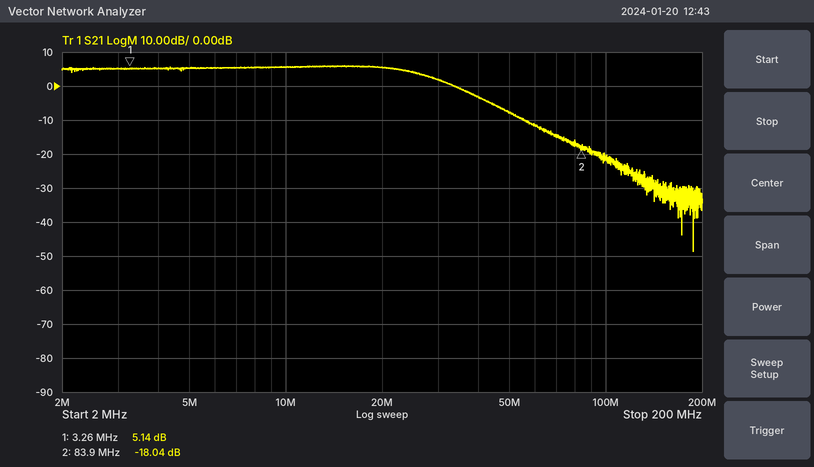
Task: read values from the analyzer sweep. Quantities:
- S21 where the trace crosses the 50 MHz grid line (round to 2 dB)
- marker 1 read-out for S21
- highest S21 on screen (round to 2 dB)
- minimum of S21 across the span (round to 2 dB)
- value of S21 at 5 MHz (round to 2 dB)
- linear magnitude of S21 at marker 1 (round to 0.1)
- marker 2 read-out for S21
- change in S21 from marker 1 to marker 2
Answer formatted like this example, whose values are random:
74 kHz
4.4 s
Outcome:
-8 dB
5.14 dB
6 dB
-48 dB
6 dB
1.8
-18.04 dB
-23.18 dB
